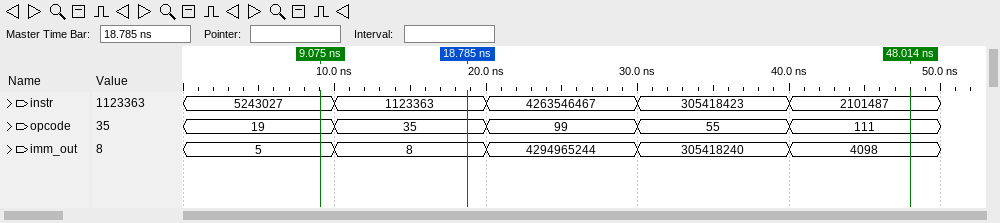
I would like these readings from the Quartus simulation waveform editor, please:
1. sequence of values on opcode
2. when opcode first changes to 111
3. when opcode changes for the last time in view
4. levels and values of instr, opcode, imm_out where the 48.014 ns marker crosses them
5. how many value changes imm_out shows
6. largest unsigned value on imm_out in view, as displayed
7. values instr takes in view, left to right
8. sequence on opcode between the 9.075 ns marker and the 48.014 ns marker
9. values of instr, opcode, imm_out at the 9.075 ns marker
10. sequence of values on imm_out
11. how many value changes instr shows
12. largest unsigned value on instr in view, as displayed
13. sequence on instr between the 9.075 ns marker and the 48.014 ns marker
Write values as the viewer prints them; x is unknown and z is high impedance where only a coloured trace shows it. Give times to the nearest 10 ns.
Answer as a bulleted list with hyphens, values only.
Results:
- 19, 35, 99, 55, 111
- 40 ns
- 40 ns
- instr=2101487, opcode=111, imm_out=4098
- 4
- 4294965244
- 5243027, 1123363, 4263546467, 305418423, 2101487
- 19, 35, 99, 55, 111
- instr=5243027, opcode=19, imm_out=5
- 5, 8, 4294965244, 305418240, 4098
- 4
- 4263546467
- 5243027, 1123363, 4263546467, 305418423, 2101487
